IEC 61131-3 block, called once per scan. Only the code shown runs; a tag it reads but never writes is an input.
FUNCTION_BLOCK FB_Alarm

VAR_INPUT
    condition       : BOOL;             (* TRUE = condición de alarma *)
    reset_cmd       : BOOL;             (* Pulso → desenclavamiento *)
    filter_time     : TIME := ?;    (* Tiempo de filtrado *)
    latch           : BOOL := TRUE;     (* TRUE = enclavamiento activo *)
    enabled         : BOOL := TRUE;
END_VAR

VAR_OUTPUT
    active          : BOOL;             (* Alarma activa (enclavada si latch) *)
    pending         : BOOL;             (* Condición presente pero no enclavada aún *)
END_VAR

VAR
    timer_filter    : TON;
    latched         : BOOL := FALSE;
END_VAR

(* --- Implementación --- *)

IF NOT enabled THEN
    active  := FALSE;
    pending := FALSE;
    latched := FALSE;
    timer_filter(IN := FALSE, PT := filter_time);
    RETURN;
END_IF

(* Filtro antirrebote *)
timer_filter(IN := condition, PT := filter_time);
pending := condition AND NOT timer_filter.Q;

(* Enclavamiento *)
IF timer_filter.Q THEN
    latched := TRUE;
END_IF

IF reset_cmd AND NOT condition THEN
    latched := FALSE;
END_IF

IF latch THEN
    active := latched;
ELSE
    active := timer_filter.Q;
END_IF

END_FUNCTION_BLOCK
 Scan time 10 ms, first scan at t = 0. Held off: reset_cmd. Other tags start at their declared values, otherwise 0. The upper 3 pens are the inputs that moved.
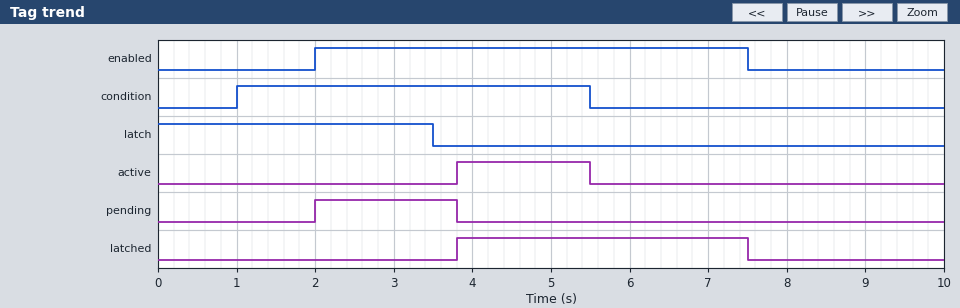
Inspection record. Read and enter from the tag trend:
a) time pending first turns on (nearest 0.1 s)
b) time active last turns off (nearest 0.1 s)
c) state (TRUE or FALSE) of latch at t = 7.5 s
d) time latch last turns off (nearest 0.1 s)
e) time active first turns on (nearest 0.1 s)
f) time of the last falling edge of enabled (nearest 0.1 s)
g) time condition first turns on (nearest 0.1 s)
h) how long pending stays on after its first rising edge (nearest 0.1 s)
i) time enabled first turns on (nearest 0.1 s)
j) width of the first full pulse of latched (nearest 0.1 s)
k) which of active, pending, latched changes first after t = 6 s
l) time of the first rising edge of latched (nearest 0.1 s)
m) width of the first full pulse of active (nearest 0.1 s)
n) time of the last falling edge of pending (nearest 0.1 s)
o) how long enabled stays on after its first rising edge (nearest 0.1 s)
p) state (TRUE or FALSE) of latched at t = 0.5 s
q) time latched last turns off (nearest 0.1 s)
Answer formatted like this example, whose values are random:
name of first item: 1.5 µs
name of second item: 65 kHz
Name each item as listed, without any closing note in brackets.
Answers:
time pending first turns on: 2.0 s
time active last turns off: 5.5 s
state (TRUE or FALSE) of latch at t = 7.5 s: FALSE
time latch last turns off: 3.5 s
time active first turns on: 3.8 s
time of the last falling edge of enabled: 7.5 s
time condition first turns on: 1.0 s
how long pending stays on after its first rising edge: 1.8 s
time enabled first turns on: 2.0 s
width of the first full pulse of latched: 3.7 s
which of active, pending, latched changes first after t = 6 s: latched
time of the first rising edge of latched: 3.8 s
width of the first full pulse of active: 1.7 s
time of the last falling edge of pending: 3.8 s
how long enabled stays on after its first rising edge: 5.5 s
state (TRUE or FALSE) of latched at t = 0.5 s: FALSE
time latched last turns off: 7.5 s
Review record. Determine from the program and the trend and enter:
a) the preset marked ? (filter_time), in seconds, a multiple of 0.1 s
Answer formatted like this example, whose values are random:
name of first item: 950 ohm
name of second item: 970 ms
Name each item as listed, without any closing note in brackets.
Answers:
the preset marked ? (filter_time), in seconds, a multiple of 0.1 s: 1.8 s
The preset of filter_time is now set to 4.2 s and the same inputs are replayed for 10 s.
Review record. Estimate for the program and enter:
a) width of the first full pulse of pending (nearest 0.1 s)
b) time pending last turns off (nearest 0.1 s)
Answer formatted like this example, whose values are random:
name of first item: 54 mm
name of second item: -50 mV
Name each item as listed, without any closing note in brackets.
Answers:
width of the first full pulse of pending: 3.5 s
time pending last turns off: 5.5 s
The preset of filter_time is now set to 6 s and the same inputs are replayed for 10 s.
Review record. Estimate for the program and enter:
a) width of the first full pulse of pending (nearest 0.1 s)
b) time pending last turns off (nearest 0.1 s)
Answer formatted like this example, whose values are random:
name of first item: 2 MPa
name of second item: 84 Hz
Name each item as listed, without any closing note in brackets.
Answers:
width of the first full pulse of pending: 3.5 s
time pending last turns off: 5.5 s
